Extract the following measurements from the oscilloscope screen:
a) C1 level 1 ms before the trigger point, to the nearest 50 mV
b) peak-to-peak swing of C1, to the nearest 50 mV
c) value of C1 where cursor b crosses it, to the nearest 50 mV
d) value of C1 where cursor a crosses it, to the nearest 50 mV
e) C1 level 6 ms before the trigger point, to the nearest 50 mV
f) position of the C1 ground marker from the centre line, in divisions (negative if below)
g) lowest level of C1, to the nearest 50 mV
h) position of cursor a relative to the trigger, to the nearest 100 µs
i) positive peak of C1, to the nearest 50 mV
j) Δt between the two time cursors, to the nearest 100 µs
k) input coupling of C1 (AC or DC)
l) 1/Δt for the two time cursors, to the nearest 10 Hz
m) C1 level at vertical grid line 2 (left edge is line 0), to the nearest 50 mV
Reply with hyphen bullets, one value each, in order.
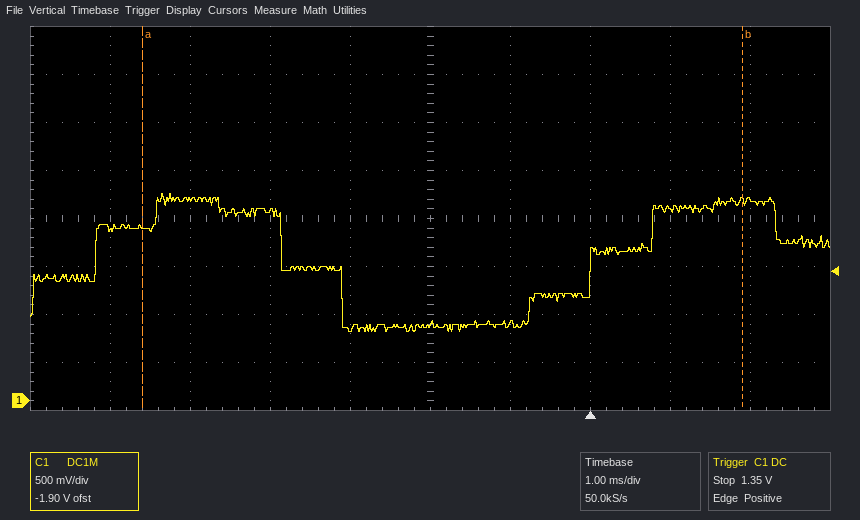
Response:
- 800 mV
- 1.45 V
- 2.10 V
- 1.80 V
- 1.80 V
- -3.8 div
- 700 mV
- -5.6 ms
- 2.15 V
- 7.5 ms
- DC
- 130 Hz
- 2.10 V
